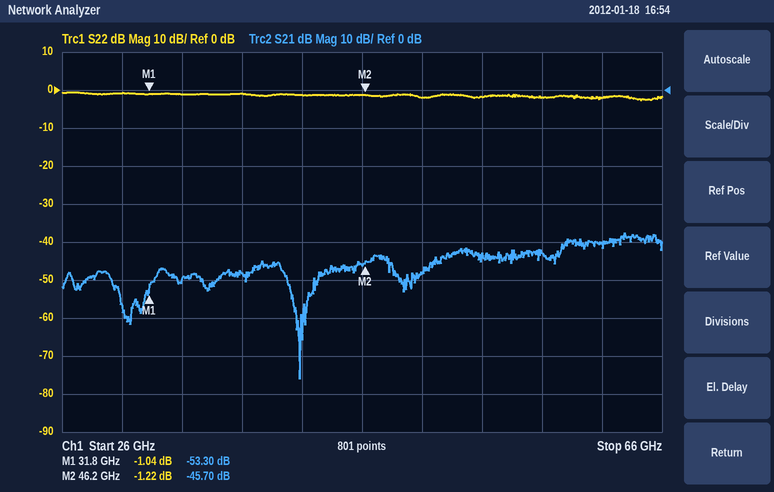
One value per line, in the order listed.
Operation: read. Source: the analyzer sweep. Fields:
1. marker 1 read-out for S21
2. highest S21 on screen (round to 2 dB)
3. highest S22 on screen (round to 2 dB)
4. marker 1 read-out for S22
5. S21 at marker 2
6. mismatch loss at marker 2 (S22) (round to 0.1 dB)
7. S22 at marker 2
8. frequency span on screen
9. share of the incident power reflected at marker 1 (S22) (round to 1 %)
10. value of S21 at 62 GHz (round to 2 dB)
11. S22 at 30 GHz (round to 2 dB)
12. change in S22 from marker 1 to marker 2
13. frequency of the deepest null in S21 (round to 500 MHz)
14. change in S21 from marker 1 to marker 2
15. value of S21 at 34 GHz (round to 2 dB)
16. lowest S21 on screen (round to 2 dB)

-53.30 dB
-38 dB
0 dB
-1.04 dB
-45.70 dB
6.1 dB
-1.22 dB
40 GHz
79 %
-40 dB
0 dB
-0.18 dB
42.0 GHz
7.60 dB
-50 dB
-76 dB
